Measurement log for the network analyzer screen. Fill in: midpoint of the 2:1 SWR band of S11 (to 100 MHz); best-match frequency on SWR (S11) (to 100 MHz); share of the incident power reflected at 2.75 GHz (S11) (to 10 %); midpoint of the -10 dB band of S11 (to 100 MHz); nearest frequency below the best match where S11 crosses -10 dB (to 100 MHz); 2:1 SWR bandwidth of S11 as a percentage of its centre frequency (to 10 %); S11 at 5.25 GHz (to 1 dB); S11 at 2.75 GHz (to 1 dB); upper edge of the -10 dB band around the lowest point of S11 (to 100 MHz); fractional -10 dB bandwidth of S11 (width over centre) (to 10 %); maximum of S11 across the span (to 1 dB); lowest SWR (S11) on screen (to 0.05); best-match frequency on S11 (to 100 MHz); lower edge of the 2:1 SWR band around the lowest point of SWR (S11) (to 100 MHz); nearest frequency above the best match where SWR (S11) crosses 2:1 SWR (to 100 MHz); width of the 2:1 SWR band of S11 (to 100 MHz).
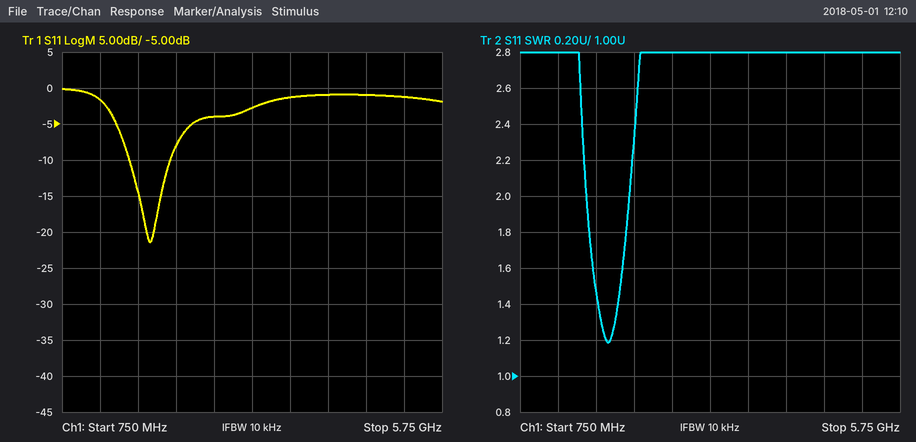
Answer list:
1.9 GHz
1.9 GHz
40 %
1.9 GHz
1.6 GHz
30 %
-1 dB
-4 dB
2.2 GHz
30 %
0 dB
1.20
1.9 GHz
1.6 GHz
2.2 GHz
600 MHz
